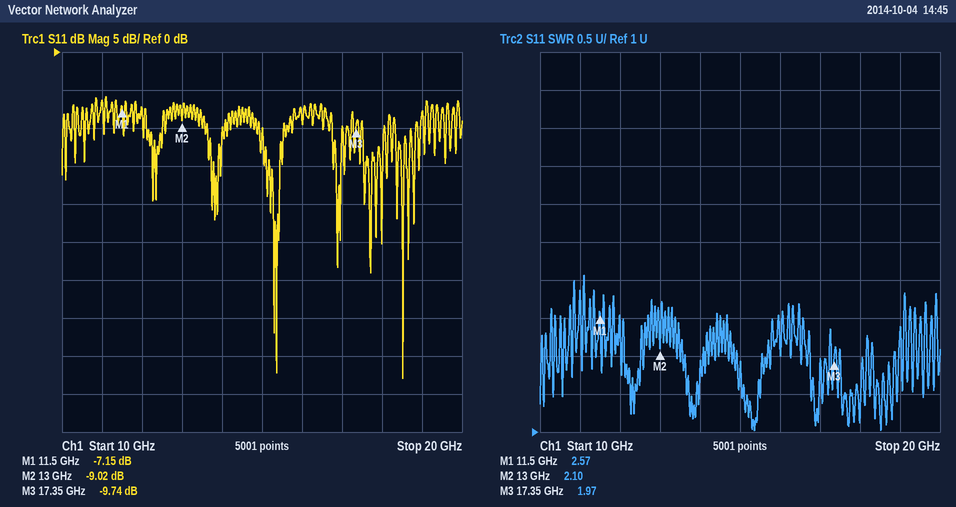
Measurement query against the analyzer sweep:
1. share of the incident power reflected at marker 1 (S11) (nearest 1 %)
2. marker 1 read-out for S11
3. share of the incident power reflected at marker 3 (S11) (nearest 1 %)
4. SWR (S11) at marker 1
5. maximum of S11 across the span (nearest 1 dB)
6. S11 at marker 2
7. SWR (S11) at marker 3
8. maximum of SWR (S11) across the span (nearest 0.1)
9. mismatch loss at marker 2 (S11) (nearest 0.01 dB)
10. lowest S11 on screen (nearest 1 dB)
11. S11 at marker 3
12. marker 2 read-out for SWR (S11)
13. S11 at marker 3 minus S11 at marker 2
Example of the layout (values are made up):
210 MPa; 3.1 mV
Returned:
19 %; -7.15 dB; 11 %; 2.57; -6 dB; -9.02 dB; 1.97; 3.1; 0.58 dB; -43 dB; -9.74 dB; 2.10; -0.72 dB
